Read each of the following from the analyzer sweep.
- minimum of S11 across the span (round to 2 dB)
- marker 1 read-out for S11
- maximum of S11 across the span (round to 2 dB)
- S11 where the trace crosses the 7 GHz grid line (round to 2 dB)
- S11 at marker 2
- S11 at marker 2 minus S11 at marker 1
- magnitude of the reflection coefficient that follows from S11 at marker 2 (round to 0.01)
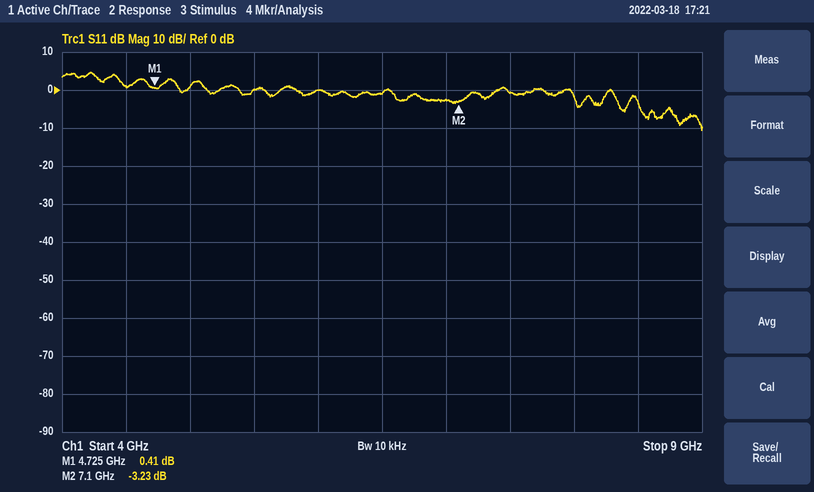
-10 dB
0.41 dB
4 dB
-2 dB
-3.23 dB
-3.64 dB
0.69
